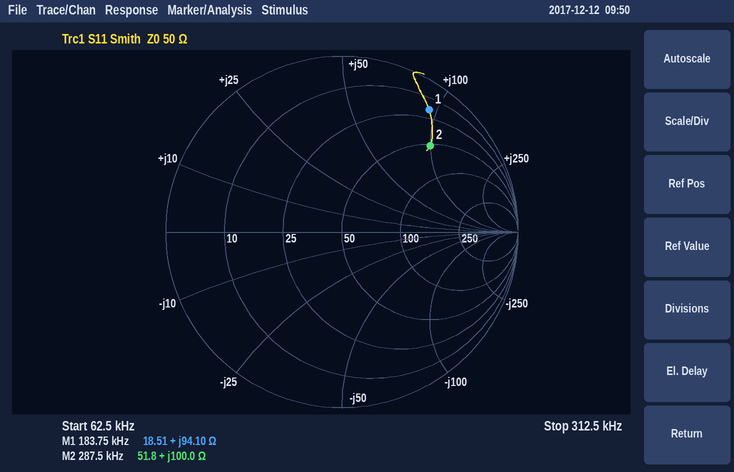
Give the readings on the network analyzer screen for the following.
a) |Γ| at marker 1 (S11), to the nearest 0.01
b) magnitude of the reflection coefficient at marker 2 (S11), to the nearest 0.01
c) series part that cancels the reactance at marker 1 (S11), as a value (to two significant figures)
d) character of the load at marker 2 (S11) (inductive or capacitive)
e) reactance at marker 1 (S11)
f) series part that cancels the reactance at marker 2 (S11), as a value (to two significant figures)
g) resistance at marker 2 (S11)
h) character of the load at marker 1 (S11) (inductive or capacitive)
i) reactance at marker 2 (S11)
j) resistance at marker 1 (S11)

0.85
0.70
9.2 nF
inductive
+94.10 Ω
5.5 nF
51.8 Ω
inductive
+100.0 Ω
18.51 Ω
